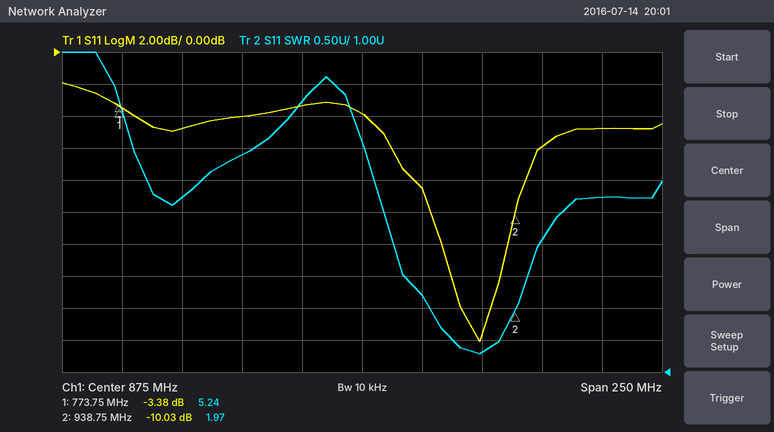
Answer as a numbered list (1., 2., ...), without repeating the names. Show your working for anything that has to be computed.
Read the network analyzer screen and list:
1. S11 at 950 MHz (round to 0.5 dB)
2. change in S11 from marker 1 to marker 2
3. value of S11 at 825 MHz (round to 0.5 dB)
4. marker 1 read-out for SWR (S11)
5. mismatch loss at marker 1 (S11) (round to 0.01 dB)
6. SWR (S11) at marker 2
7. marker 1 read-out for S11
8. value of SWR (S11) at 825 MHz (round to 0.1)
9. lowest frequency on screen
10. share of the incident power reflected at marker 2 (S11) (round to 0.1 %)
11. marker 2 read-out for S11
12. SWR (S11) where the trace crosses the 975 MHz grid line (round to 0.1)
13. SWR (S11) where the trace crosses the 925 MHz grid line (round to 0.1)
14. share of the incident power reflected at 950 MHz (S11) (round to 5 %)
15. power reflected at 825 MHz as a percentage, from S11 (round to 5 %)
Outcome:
1. -6.0 dB
2. -10.03 − (-3.38) = -6.65 dB
3. -4.0 dB
4. 5.24
5. −10 log10(1 − 10^(-3.38/10)) ≈ 2.67 dB
6. 1.97
7. -3.38 dB
8. 4.4
9. 750 MHz
10. 10^(-10.03/10) ≈ 9.9 %
11. -10.03 dB
12. 3.7
13. 1.3
14. 10^(-6/10) ≈ 25 %
15. 10^(-4/10) ≈ 40 %
